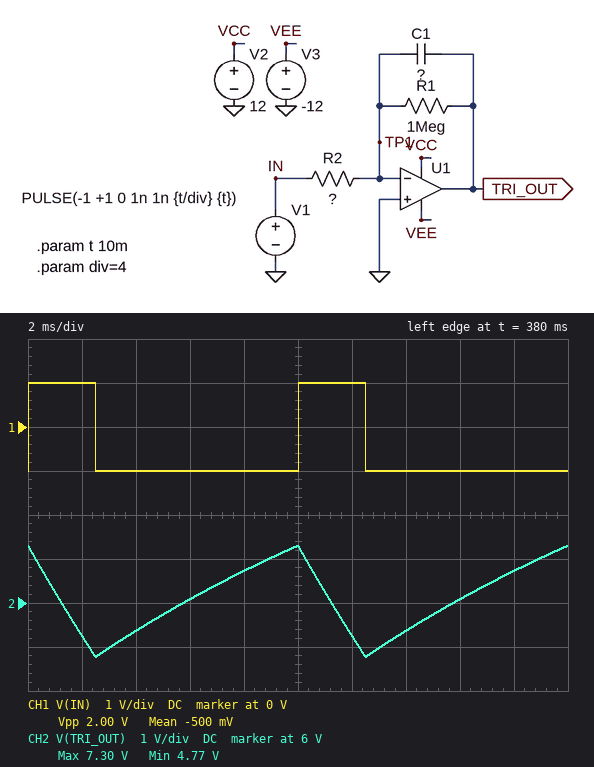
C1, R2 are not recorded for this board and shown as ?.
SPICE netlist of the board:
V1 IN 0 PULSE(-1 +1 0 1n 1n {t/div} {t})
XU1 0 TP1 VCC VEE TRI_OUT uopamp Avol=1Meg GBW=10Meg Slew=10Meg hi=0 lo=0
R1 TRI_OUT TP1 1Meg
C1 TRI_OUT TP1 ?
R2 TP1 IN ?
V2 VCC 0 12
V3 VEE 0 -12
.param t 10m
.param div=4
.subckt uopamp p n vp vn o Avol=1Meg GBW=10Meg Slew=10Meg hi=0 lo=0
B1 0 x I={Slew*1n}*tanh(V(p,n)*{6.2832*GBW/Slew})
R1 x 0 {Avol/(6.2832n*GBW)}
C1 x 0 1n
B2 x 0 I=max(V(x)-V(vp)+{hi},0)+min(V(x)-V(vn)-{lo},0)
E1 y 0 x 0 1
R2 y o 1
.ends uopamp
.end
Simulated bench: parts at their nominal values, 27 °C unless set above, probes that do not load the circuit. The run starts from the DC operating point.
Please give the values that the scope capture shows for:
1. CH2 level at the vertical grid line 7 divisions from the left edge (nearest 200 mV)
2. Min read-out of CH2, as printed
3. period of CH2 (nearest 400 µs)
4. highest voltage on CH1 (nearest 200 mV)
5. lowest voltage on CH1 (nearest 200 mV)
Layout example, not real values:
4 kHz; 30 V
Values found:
5.4 V; 4.77 V; 10.0 ms; 1.0 V; -1.0 V
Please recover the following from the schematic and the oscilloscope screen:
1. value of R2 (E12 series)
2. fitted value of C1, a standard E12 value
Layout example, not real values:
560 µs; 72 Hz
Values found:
82 kΩ; 18 nF
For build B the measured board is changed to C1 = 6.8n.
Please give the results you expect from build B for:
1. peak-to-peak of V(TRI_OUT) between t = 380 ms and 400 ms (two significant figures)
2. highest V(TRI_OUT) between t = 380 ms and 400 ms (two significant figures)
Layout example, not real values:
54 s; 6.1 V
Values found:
6.5 V; 9.0 V
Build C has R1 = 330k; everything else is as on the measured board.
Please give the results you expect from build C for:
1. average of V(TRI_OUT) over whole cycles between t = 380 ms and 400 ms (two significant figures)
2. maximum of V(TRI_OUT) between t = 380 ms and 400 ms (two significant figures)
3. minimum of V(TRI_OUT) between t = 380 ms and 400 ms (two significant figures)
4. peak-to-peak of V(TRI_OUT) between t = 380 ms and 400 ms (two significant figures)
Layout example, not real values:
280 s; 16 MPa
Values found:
2.0 V; 3.1 V; 630 mV; 2.4 V
